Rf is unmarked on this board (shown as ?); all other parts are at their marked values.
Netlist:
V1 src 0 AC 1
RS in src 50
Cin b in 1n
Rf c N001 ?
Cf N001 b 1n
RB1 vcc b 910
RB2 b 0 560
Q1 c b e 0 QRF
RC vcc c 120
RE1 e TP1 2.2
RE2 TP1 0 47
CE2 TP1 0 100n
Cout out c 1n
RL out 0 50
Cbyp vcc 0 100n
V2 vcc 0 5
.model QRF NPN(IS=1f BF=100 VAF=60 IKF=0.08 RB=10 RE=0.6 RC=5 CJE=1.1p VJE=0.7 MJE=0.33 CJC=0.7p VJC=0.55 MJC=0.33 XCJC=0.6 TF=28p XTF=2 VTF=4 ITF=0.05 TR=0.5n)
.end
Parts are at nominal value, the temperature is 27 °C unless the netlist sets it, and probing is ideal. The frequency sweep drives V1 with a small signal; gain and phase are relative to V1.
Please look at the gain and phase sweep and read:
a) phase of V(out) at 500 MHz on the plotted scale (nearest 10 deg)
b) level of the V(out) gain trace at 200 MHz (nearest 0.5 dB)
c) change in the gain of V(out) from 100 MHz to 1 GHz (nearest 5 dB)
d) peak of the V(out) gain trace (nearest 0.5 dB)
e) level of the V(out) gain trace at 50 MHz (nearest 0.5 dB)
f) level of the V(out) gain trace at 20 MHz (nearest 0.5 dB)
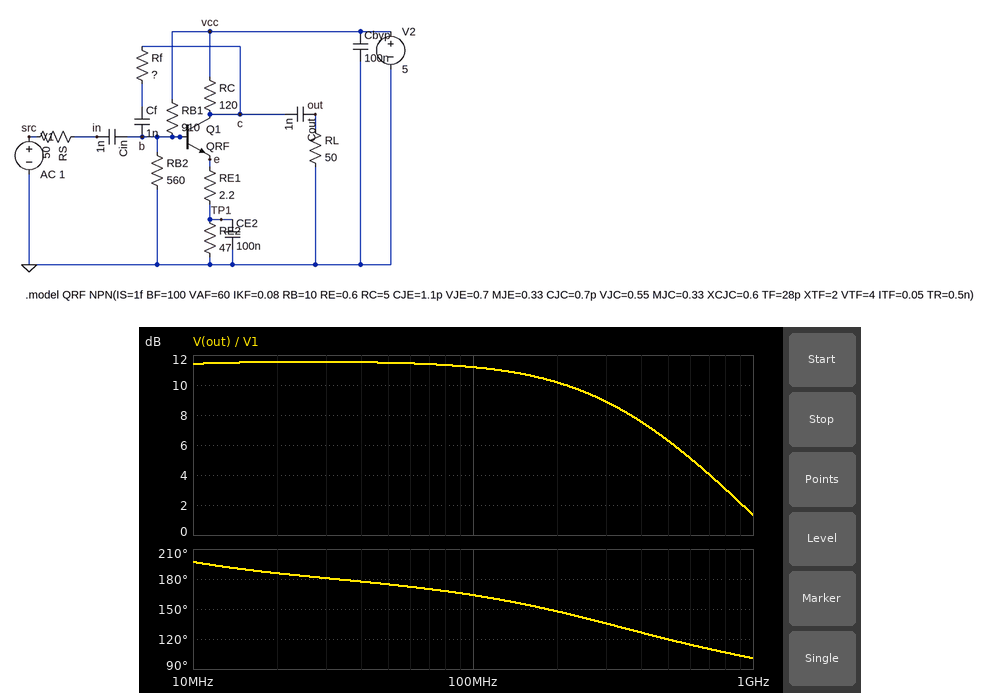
120 deg
10.0 dB
-10 dB
11.5 dB
11.5 dB
11.5 dB
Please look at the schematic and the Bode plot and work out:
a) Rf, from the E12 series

680 Ω
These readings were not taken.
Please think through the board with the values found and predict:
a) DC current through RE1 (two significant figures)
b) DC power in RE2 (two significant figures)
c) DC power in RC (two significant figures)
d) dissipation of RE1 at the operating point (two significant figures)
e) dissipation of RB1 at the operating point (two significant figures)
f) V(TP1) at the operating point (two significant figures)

20 mA
20 mW
49 mW
920 µW
11 mW
960 mV
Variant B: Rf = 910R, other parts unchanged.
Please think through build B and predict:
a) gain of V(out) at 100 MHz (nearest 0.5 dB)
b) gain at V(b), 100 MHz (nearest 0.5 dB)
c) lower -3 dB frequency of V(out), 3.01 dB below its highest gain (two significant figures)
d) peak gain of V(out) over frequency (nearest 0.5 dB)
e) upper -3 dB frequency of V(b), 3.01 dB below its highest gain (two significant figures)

12.0 dB
-5.5 dB
2.3 MHz
12.5 dB
330 MHz
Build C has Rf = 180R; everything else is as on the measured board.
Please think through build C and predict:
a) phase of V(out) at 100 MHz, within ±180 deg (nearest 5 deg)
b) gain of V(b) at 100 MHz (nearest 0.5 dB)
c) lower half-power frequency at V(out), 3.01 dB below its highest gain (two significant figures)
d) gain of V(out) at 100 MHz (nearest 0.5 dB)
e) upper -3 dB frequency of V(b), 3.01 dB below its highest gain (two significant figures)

170 deg
-10.5 dB
3.5 MHz
5.5 dB
1.0 GHz
